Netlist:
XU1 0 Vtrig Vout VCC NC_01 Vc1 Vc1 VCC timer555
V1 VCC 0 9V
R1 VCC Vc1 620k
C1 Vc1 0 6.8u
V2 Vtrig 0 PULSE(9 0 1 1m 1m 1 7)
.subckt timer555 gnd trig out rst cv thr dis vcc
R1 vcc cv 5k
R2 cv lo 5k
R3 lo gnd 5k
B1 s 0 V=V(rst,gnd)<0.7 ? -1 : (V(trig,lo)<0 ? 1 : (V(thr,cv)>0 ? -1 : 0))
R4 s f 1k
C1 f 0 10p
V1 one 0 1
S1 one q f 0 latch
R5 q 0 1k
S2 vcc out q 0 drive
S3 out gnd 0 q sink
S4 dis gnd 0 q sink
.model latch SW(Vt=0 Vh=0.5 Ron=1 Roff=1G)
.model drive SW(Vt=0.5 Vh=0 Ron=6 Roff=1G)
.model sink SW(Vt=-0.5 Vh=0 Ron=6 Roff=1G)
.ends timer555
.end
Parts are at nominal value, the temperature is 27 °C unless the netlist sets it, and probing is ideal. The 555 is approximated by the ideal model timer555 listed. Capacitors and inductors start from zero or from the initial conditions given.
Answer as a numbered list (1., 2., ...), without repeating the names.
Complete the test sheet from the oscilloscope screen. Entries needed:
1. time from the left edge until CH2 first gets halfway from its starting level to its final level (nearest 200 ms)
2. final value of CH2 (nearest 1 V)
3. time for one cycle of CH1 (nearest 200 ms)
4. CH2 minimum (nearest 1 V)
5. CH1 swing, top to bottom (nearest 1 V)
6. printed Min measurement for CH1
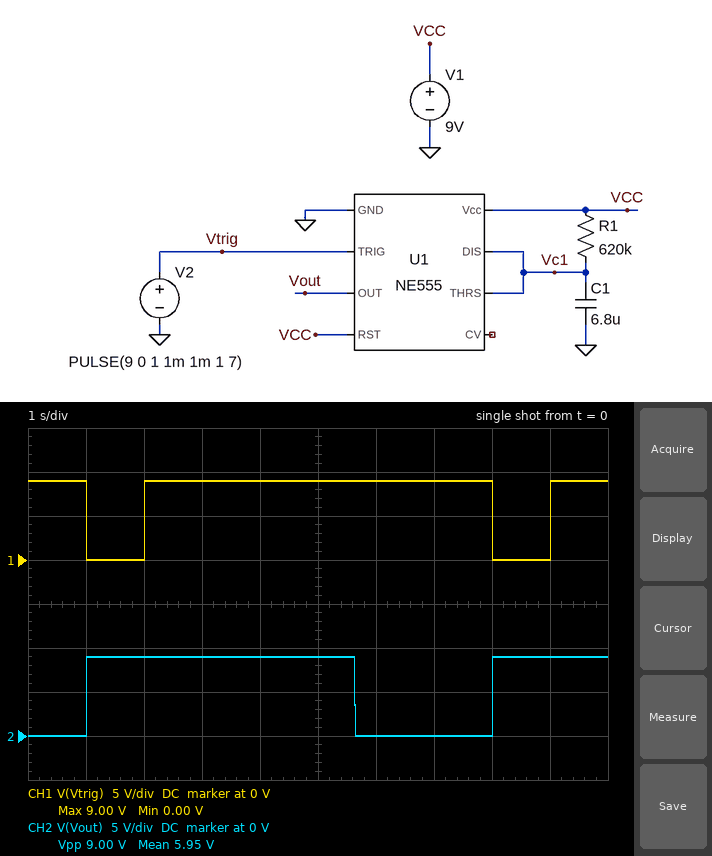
1. 1.0 s
2. 9 V
3. 7.0 s
4. 0 V
5. 9 V
6. 0.00 V
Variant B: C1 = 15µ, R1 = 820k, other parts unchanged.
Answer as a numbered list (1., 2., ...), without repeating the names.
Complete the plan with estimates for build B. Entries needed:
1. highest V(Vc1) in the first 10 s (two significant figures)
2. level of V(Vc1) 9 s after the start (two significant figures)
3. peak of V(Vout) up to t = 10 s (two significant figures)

1. 4.7 V
2. 4.3 V
3. 9.0 V
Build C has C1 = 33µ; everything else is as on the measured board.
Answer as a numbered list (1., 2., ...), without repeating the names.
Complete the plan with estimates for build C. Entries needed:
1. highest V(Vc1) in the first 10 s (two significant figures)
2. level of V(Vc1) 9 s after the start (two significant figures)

1. 3.2 V
2. 2.9 V
